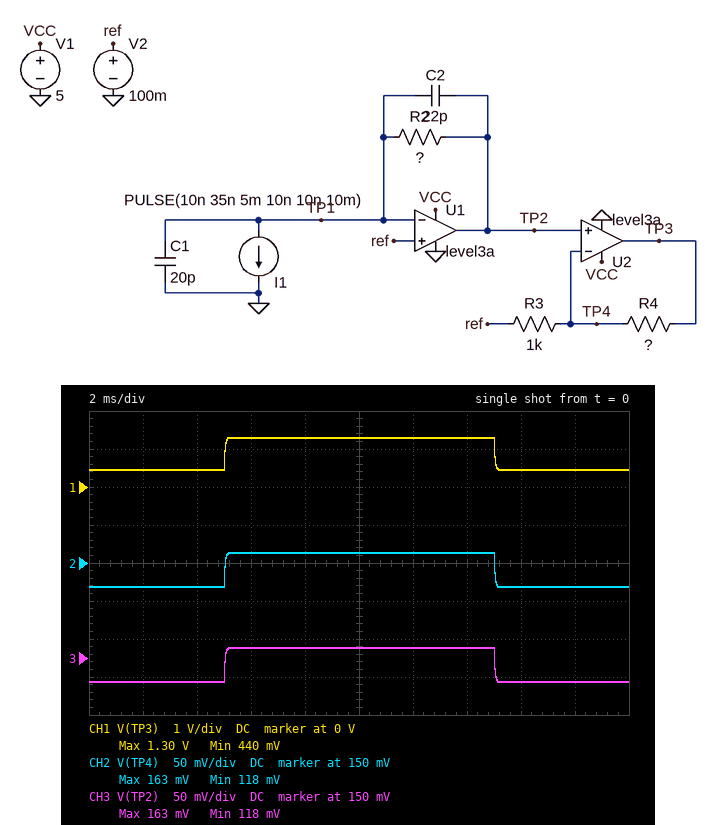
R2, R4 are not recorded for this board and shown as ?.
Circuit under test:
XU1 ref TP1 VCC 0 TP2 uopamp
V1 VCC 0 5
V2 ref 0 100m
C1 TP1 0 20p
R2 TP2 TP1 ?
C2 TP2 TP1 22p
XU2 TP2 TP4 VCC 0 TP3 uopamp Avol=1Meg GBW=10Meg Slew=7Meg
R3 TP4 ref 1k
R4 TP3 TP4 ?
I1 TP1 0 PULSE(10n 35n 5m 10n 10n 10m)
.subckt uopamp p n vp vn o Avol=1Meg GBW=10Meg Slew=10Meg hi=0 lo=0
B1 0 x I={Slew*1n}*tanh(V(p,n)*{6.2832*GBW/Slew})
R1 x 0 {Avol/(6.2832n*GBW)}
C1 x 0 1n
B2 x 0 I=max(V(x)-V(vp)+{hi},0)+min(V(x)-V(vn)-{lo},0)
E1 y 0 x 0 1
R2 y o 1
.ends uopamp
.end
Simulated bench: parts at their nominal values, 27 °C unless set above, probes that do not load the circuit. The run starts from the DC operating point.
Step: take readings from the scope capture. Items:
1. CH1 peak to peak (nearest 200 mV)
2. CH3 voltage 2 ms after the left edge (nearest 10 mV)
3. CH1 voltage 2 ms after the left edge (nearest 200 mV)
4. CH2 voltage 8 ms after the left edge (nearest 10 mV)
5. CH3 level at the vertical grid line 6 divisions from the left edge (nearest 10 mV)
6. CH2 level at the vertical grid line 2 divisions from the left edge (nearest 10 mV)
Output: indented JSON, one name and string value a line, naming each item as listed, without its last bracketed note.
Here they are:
{
  "CH1 peak to peak": "800 mV",
  "CH3 voltage 2 ms after the left edge": "120 mV",
  "CH1 voltage 2 ms after the left edge": "400 mV",
  "CH2 voltage 8 ms after the left edge": "160 mV",
  "CH3 level at the vertical grid line 6 divisions from the left edge": "160 mV",
  "CH2 level at the vertical grid line 2 divisions from the left edge": "120 mV"
}
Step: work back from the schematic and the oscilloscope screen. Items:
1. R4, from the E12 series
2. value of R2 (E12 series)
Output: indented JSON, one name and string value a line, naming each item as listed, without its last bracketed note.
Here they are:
{
  "R4, from the E12 series": "18 kΩ",
  "value of R2": "1.8 MΩ"
}
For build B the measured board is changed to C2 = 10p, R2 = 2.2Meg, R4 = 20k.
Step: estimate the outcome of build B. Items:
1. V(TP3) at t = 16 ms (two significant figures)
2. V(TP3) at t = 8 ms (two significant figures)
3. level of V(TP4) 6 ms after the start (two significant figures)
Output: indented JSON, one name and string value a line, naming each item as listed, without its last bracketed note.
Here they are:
{
  "V(TP3) at t = 16 ms": "560 mV",
  "V(TP3) at t = 8 ms": "1.7 V",
  "level of V(TP4) 6 ms after the start": "180 mV"
}
